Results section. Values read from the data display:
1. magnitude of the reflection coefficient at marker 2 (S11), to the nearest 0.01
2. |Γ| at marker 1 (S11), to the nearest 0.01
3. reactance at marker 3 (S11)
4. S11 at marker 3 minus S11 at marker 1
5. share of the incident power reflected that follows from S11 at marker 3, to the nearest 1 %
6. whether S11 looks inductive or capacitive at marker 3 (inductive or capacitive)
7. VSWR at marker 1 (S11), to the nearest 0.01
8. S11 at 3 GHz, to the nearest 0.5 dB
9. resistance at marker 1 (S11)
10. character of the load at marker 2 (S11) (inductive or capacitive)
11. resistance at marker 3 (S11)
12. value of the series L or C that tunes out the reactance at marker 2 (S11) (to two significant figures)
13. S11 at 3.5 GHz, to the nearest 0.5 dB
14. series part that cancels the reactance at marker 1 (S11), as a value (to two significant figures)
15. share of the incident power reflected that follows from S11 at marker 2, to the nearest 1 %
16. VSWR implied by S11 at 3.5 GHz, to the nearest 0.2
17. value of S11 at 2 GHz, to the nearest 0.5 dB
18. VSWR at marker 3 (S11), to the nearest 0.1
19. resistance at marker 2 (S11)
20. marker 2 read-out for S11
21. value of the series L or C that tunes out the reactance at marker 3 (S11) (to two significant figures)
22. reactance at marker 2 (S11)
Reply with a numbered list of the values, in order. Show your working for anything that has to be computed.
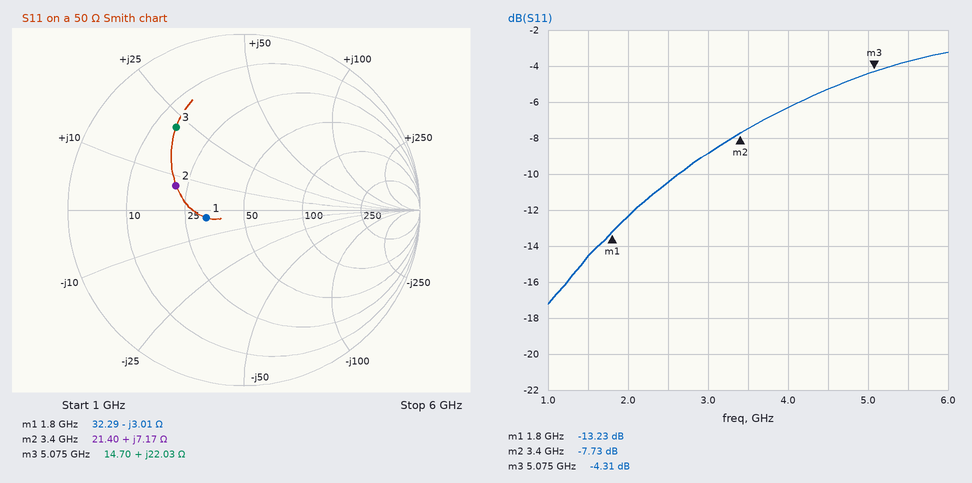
1. 0.41
2. 0.22
3. +22.03 Ω
4. -4.31 − (-13.23) = 8.92 dB
5. 10^(-4.31/10) ≈ 37 %
6. inductive
7. (1 + 0.2180)/(1 − 0.2180) ≈ 1.56
8. -9.0 dB
9. 32.29 Ω
10. inductive
11. 14.70 Ω
12. C = 1/(2π × 3.4 GHz × 7.17 Ω) ≈ 6.5 pF
13. -7.5 dB
14. L = 3.01 Ω/(2π × 1.8 GHz) ≈ 266 pH, so 270 pH to two significant figures
15. 10^(-7.73/10) ≈ 17 %
16. |Γ| = 10^(-7.5/20) = 0.4217; VSWR = (1 + 0.4217)/(1 − 0.4217) ≈ 2.46, so 2.4 to the nearest 0.2
17. -12.5 dB
18. 4.1
19. 21.40 Ω
20. -7.73 dB
21. C = 1/(2π × 5.075 GHz × 22.03 Ω) ≈ 1.4 pF
22. +7.17 Ω
